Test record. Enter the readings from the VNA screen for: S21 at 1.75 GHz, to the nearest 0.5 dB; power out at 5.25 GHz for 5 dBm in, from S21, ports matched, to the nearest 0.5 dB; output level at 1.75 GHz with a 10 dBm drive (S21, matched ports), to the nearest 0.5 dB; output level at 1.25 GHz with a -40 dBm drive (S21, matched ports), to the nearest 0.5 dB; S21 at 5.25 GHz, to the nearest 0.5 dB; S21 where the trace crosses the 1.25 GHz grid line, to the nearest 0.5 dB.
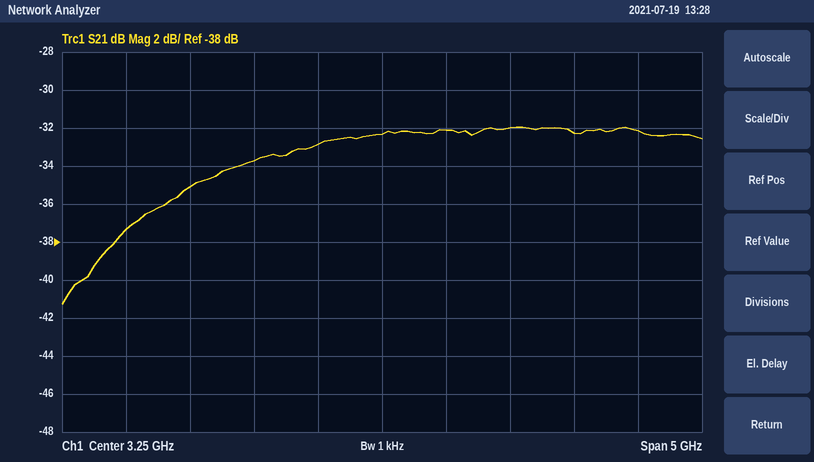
-35.0 dB
-27.0 dBm
-25.0 dBm
-77.5 dBm
-32.0 dB
-37.5 dB
